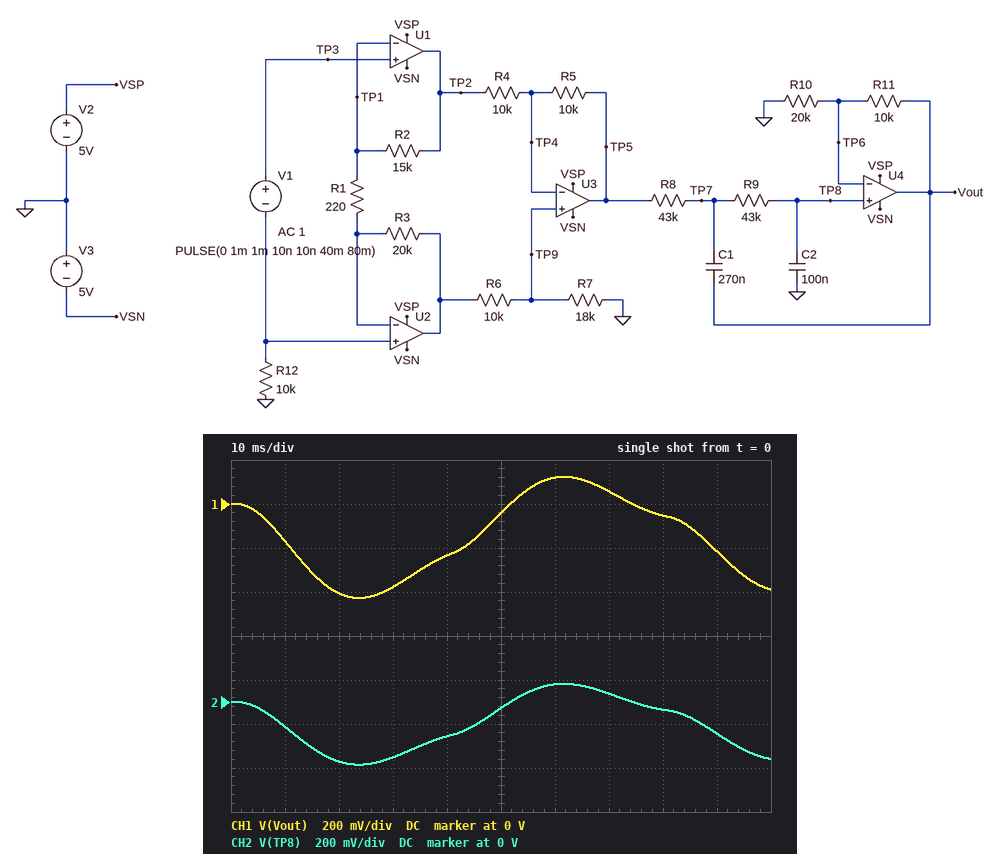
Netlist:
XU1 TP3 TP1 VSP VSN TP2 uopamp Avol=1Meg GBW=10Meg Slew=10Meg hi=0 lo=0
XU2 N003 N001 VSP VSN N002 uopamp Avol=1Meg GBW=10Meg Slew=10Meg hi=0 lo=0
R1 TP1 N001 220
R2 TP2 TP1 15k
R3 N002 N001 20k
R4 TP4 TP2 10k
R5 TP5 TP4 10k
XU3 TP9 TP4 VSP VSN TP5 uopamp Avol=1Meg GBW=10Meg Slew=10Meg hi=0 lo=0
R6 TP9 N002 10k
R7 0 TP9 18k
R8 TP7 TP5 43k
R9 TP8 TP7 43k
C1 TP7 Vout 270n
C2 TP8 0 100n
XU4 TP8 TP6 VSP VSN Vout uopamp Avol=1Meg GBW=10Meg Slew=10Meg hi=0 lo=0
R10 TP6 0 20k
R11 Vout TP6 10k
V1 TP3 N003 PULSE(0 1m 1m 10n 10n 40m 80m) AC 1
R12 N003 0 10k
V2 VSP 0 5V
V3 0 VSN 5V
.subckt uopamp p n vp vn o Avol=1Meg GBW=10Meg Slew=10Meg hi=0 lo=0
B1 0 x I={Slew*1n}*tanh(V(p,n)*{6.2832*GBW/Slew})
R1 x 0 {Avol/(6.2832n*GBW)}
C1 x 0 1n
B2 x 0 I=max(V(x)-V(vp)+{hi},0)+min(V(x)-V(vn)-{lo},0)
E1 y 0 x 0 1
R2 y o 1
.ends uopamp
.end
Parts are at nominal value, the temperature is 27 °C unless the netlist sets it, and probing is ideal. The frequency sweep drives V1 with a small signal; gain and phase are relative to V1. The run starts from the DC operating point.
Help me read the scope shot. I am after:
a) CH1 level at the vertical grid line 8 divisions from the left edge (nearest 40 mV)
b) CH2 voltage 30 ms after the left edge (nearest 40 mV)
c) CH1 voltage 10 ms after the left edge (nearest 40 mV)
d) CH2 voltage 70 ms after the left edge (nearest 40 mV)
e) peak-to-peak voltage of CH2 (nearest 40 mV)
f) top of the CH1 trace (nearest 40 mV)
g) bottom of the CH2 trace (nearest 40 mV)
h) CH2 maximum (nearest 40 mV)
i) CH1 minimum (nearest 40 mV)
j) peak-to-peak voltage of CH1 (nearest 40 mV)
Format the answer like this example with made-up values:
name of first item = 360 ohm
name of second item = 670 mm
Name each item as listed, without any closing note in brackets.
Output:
CH1 level at the vertical grid line 8 divisions from the left edge = -40 mV
CH2 voltage 30 ms after the left edge = -240 mV
CH1 voltage 10 ms after the left edge = -160 mV
CH2 voltage 70 ms after the left edge = 40 mV
peak-to-peak voltage of CH2 = 360 mV
top of the CH1 trace = 120 mV
bottom of the CH2 trace = -280 mV
CH2 maximum = 80 mV
CH1 minimum = -440 mV
peak-to-peak voltage of CH1 = 560 mV
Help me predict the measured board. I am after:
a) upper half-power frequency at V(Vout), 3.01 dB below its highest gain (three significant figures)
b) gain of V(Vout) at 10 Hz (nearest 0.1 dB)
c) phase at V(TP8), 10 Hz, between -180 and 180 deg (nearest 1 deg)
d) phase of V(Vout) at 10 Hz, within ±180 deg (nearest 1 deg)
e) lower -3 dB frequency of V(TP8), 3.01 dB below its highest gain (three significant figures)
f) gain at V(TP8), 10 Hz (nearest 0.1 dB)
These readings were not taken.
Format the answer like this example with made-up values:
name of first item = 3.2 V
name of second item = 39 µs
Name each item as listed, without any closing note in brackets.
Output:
upper half-power frequency at V(Vout), 3.01 dB below its highest gain = 25.8 Hz
gain of V(Vout) at 10 Hz = 50.6 dB
phase at V(TP8), 10 Hz, between -180 and 180 deg = 168 deg
phase of V(Vout) at 10 Hz, within ±180 deg = 168 deg
lower -3 dB frequency of V(TP8), 3.01 dB below its highest gain = 16.5 Hz
gain at V(TP8), 10 Hz = 47.1 dB
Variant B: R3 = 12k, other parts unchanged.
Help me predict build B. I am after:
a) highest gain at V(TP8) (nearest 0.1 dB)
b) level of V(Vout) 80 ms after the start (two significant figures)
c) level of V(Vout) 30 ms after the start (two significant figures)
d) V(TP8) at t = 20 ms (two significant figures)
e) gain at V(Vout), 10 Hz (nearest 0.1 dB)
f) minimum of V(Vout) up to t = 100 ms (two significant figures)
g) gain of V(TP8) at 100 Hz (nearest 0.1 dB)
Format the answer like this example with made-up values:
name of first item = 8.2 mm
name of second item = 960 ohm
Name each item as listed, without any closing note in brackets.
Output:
highest gain at V(TP8) = 51.1 dB
level of V(Vout) 80 ms after the start = -40 mV
level of V(Vout) 30 ms after the start = -280 mV
V(TP8) at t = 20 ms = -200 mV
gain at V(Vout), 10 Hz = 48.1 dB
minimum of V(Vout) up to t = 100 ms = -320 mV
gain of V(TP8) at 100 Hz = 17.4 dB
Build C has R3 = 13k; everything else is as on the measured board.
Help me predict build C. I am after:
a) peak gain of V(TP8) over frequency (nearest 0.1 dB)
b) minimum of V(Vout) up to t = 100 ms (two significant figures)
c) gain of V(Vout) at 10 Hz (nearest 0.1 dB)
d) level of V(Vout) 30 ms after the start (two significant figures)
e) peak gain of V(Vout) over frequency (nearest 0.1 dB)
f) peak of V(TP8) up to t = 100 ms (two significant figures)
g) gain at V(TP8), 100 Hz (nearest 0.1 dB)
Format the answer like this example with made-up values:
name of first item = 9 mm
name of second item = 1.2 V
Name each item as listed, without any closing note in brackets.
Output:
peak gain of V(TP8) over frequency = 51.5 dB
minimum of V(Vout) up to t = 100 ms = -330 mV
gain of V(Vout) at 10 Hz = 48.5 dB
level of V(Vout) 30 ms after the start = -290 mV
peak gain of V(Vout) over frequency = 55.0 dB
peak of V(TP8) up to t = 100 ms = 64 mV
gain at V(TP8), 100 Hz = 17.8 dB
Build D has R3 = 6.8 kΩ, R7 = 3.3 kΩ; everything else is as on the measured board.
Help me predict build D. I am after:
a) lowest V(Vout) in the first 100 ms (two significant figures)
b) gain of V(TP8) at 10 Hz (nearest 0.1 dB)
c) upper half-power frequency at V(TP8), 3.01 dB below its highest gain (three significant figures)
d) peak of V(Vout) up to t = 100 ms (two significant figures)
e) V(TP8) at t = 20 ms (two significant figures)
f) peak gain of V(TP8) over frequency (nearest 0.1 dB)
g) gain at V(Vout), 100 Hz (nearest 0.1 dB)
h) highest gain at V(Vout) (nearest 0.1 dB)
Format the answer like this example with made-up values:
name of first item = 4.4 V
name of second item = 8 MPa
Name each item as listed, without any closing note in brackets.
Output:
lowest V(Vout) in the first 100 ms = -190 mV
gain of V(TP8) at 10 Hz = 40.2 dB
upper half-power frequency at V(TP8), 3.01 dB below its highest gain = 25.8 Hz
peak of V(Vout) up to t = 100 ms = 56 mV
V(TP8) at t = 20 ms = -120 mV
peak gain of V(TP8) over frequency = 46.8 dB
gain at V(Vout), 100 Hz = 16.6 dB
highest gain at V(Vout) = 50.3 dB
